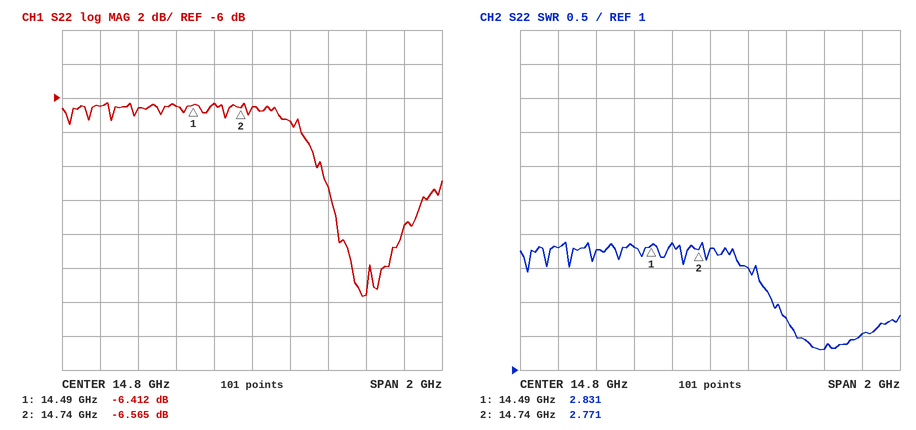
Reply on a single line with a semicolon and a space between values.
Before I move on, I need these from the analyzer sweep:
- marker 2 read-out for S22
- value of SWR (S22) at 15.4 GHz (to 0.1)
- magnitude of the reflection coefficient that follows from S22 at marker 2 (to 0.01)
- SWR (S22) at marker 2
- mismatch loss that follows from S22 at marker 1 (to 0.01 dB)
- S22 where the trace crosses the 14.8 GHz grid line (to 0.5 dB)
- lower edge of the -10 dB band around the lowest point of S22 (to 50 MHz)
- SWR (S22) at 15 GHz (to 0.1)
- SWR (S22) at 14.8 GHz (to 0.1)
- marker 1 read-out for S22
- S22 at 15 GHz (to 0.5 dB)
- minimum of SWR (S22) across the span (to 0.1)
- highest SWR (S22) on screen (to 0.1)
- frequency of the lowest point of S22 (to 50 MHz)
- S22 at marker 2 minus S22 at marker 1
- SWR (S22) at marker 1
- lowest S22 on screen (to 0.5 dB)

-6.565 dB; 1.3; 0.47; 2.771; 1.13 dB; -6.5 dB; 15.15 GHz; 2.5; 2.8; -6.412 dB; -7.5 dB; 1.3; 2.9; 15.40 GHz; -0.153 dB; 2.831; -17.5 dB
